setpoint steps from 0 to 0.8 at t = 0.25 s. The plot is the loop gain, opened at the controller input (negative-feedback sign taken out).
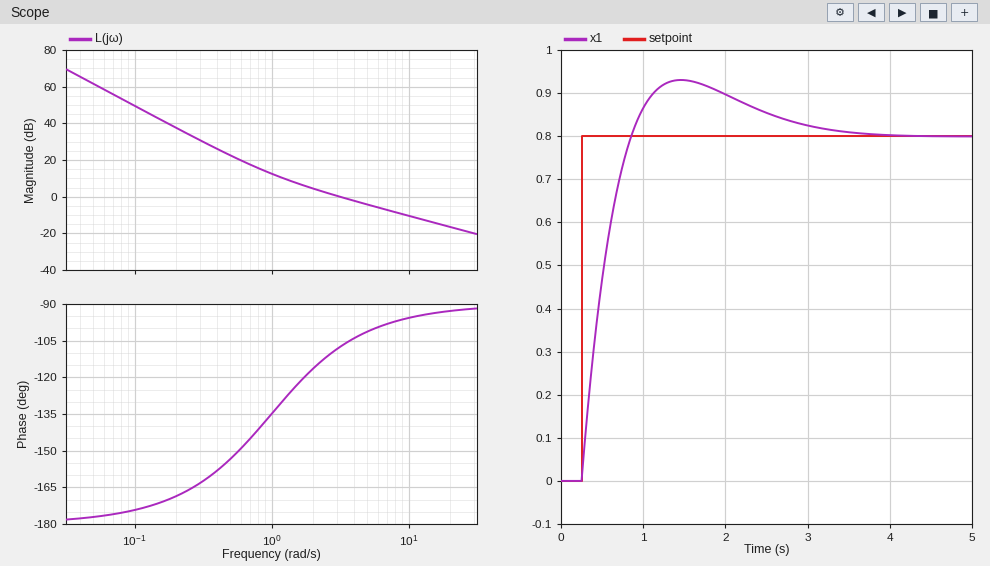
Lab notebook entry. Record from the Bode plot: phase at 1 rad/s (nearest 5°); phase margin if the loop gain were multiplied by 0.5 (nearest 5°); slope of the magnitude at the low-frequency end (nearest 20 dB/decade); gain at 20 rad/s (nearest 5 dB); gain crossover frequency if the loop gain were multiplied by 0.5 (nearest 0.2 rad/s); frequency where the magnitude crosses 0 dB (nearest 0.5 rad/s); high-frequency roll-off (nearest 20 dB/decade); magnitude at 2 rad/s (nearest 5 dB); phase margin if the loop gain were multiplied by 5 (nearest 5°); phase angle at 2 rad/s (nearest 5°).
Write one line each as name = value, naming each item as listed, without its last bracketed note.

phase at 1 rad/s = -135°
phase margin if the loop gain were multiplied by 0.5 = 60°
slope of the magnitude at the low-frequency end = -40 dB/decade
gain at 20 rad/s = -15 dB
gain crossover frequency if the loop gain were multiplied by 0.5 = 1.8 rad/s
frequency where the magnitude crosses 0 dB = 3.0 rad/s
high-frequency roll-off = -20 dB/decade
magnitude at 2 rad/s = 5 dB
phase margin if the loop gain were multiplied by 5 = 85°
phase angle at 2 rad/s = -115°
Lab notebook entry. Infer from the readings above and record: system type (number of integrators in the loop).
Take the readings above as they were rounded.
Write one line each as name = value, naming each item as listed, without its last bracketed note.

system type = 2
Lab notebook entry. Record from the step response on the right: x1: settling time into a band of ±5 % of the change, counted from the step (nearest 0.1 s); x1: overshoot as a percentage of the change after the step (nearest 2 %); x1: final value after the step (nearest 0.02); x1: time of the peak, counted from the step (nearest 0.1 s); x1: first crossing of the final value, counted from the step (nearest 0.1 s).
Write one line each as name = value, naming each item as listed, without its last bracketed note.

x1: settling time into a band of ±5 % of the change, counted from the step = 2.5 s
x1: overshoot as a percentage of the change after the step = 16 %
x1: final value after the step = 0.80
x1: time of the peak, counted from the step = 1.2 s
x1: first crossing of the final value, counted from the step = 0.6 s
